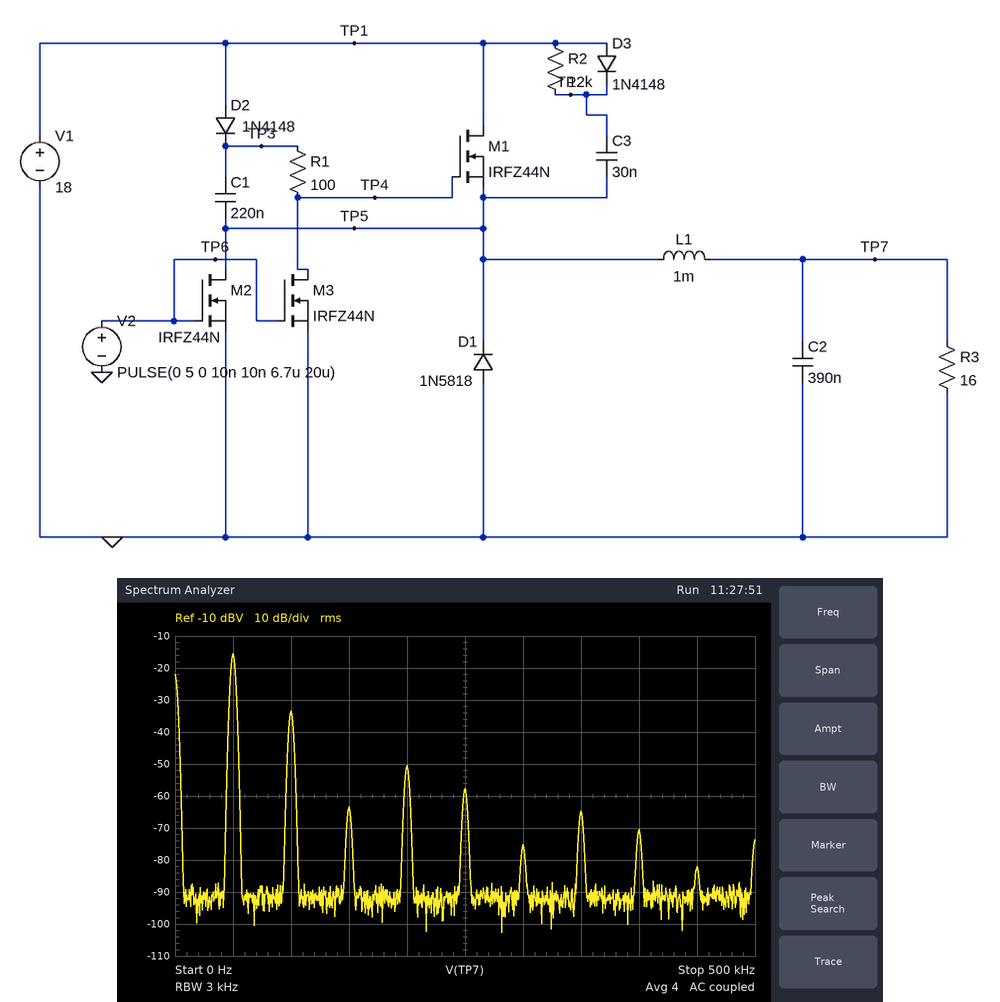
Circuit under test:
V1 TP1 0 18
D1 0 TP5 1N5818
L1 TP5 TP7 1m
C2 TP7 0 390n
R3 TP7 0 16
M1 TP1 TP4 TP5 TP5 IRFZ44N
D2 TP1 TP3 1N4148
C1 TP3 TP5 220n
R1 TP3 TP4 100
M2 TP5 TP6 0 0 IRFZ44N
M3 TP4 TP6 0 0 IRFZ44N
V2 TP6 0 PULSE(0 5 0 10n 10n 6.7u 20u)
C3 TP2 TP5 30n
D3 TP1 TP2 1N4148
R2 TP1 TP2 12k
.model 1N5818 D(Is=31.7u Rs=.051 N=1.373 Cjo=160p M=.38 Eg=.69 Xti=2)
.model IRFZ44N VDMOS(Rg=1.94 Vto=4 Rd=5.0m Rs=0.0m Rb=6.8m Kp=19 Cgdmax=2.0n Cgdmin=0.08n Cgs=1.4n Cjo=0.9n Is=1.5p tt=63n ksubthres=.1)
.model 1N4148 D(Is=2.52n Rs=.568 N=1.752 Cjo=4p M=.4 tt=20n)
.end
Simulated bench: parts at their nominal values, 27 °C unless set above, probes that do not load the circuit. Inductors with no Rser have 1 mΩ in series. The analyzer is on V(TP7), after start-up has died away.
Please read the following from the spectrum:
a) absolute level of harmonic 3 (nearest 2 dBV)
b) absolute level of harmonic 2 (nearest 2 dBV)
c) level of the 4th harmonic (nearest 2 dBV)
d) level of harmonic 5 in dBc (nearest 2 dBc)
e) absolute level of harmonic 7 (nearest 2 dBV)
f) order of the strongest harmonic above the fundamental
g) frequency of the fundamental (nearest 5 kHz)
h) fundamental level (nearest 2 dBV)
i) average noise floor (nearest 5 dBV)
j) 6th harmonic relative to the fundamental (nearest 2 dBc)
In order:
-64 dBV
-34 dBV
-50 dBV
-42 dBc
-64 dBV
2
50 kHz
-16 dBV
-90 dBV
-60 dBc
